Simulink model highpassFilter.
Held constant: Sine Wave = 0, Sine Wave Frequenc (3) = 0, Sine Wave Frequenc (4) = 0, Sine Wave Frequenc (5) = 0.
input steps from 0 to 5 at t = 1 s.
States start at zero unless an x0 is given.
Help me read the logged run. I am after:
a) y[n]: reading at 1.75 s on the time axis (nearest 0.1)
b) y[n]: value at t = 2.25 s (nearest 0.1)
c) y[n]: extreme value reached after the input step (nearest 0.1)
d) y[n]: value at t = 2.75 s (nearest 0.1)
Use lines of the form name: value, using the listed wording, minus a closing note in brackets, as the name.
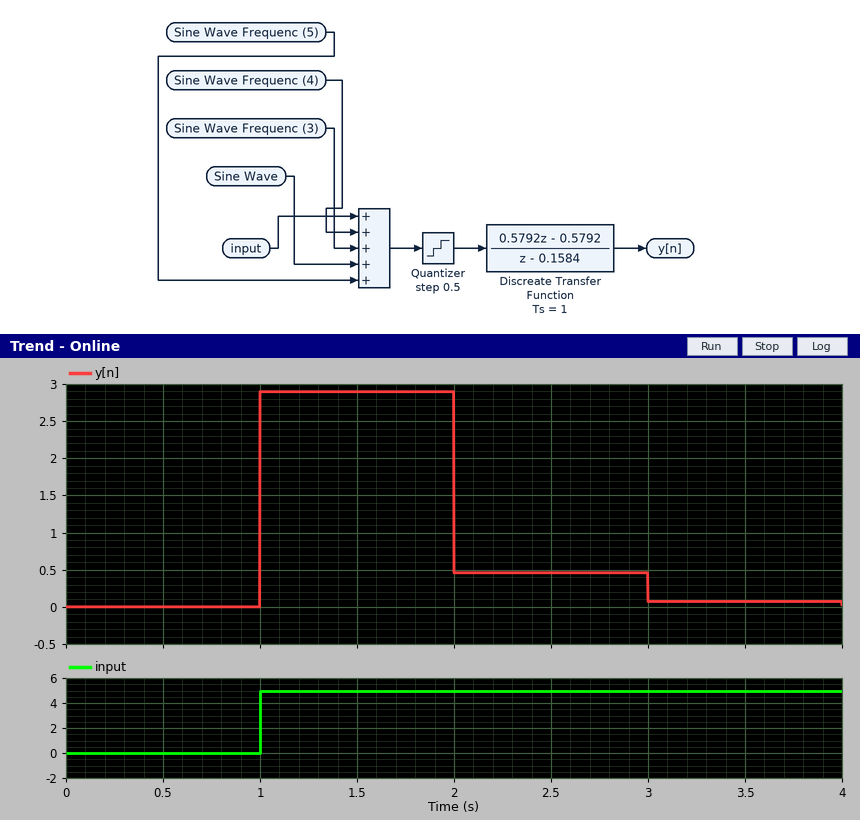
y[n]: reading at 1.75 s on the time axis: 2.9
y[n]: value at t = 2.25 s: 0.5
y[n]: extreme value reached after the input step: 2.9
y[n]: value at t = 2.75 s: 0.5
